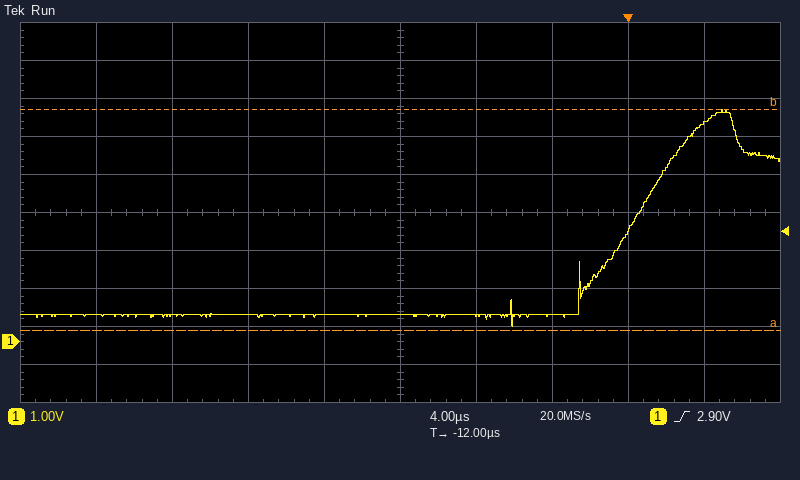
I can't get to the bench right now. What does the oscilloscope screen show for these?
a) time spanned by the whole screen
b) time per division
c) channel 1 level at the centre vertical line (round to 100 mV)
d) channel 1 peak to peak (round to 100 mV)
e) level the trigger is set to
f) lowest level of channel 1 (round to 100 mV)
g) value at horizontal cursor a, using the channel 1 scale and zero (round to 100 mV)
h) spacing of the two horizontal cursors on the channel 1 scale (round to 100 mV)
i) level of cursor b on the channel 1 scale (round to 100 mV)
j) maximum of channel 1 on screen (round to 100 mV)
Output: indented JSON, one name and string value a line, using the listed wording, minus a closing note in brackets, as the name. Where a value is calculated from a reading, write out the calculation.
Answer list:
{
  "time spanned by the whole screen": "40 µs",
  "time per division": "4 µs",
  "channel 1 level at the centre vertical line": "700 mV",
  "channel 1 peak to peak": "6.1 V − (400 mV) = 5.7 V",
  "level the trigger is set to": "2.90 V",
  "lowest level of channel 1": "400 mV",
  "value at horizontal cursor a, using the channel 1 scale and zero": "300 mV",
  "spacing of the two horizontal cursors on the channel 1 scale": "5.8 V",
  "level of cursor b on the channel 1 scale": "6.1 V",
  "maximum of channel 1 on screen": "6.1 V"
}
